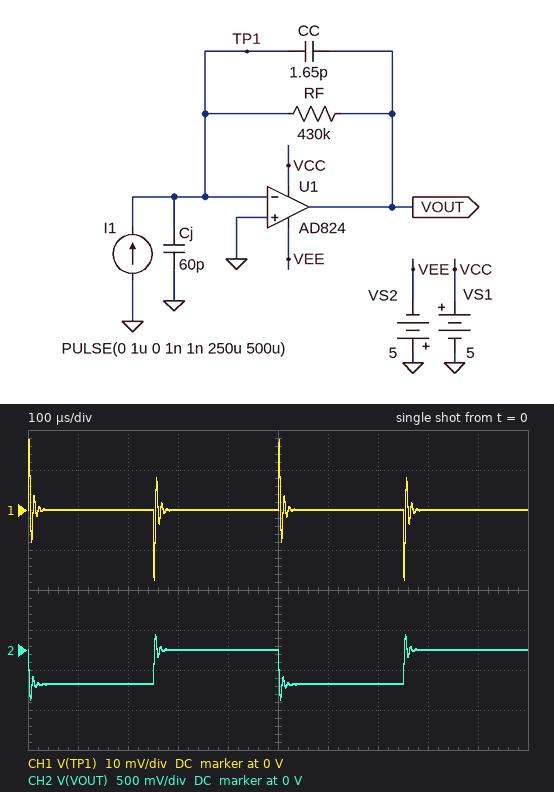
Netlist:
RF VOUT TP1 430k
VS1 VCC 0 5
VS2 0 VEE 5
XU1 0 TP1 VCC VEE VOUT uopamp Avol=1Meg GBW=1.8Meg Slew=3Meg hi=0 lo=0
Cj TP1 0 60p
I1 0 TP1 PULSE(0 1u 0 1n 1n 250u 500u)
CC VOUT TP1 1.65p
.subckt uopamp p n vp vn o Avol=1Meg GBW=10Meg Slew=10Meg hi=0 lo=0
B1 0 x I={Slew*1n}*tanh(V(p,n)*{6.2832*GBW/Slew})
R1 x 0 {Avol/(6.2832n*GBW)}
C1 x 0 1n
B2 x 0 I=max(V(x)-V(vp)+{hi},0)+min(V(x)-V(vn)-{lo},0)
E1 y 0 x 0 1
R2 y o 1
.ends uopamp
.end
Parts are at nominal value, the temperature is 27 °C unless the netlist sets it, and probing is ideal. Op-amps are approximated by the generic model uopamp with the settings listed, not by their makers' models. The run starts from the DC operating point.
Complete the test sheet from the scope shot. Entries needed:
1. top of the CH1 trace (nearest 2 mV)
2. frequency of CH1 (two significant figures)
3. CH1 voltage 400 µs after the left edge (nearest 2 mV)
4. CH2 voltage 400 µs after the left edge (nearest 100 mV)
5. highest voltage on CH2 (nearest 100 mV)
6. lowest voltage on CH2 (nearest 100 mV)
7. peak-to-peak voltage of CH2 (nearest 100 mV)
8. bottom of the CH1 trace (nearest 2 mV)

18 mV
4.0 kHz
0 V
0 V
200 mV
-600 mV
800 mV
-18 mV
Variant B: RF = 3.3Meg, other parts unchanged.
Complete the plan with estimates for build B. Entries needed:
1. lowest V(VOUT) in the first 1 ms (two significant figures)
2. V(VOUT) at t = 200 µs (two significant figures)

-3.5 V
-3.3 V
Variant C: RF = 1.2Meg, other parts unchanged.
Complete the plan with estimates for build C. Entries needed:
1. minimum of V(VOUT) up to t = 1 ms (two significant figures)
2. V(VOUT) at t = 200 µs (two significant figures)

-1.5 V
-1.2 V
